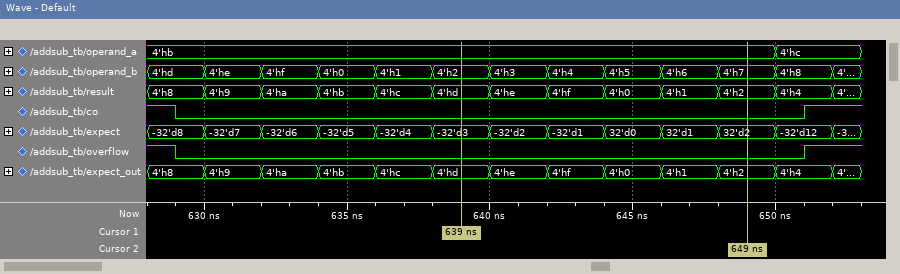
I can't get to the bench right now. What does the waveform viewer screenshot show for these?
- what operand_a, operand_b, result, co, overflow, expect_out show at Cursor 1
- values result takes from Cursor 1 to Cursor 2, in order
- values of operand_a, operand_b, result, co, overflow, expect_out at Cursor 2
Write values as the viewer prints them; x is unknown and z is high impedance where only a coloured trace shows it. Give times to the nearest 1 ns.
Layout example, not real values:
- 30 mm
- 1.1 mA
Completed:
- operand_a=4'hb, operand_b=4'h2, result=4'hd, co=0, overflow=0, expect_out=4'hd
- 4'hd, 4'he, 4'hf, 4'h0, 4'h1, 4'h2
- operand_a=4'hb, operand_b=4'h7, result=4'h2, co=0, overflow=0, expect_out=4'h2
